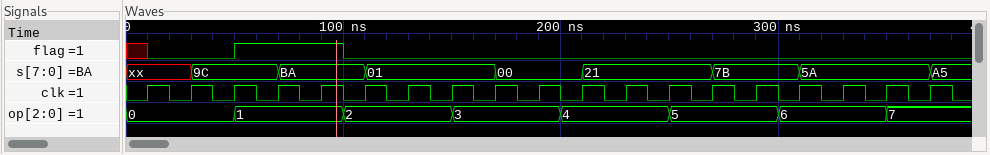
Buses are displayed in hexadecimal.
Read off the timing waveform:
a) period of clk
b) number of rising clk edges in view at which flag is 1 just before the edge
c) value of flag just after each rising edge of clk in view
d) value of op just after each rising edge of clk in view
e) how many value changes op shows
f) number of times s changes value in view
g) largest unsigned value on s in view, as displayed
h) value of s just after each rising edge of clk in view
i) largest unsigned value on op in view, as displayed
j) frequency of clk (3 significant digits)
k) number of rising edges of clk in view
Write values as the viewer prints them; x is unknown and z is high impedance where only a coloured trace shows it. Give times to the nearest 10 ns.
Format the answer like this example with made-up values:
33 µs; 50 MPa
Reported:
20 ns; 2; 0 0 1 1 1 0 0 0 0 0 0 0 0 0 0 0 0 0 0; 0, 0, 1, 1, 1, 2, 2, 3, 3, 3, 4, 4, 5, 5, 5, 6, 6, 7, 7; 7; 8; BA; xx, 9C, 9C, BA, BA, 01, 01, 01, 00, 00, 21, 21, 21, 7B, 7B, 5A, 5A, 5A, A5; 7; 50.0 MHz; 19
